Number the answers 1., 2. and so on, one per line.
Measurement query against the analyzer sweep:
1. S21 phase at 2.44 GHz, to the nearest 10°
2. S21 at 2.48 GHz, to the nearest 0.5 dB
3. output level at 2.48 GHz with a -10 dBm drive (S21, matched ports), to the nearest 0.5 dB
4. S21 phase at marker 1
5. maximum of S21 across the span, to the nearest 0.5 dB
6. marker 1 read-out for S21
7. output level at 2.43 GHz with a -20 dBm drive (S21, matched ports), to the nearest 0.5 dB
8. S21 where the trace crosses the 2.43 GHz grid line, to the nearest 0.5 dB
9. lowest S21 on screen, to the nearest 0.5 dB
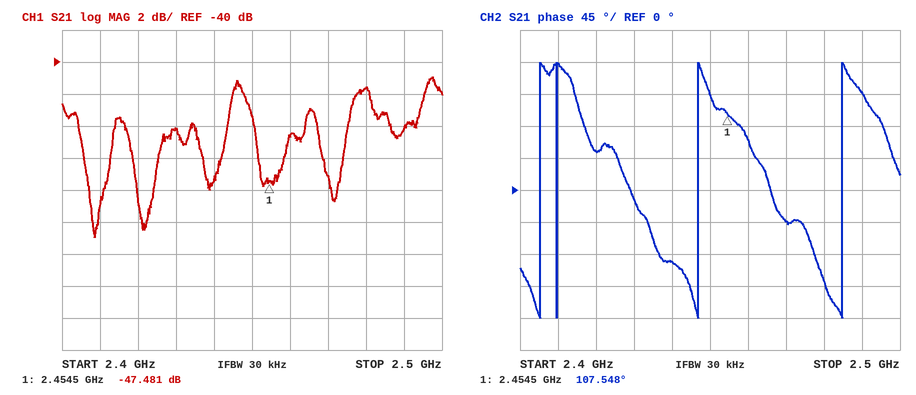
1. -100°
2. -41.5 dB
3. -51.5 dBm
4. 107.548°
5. -41.0 dB
6. -47.481 dB
7. -64.0 dBm
8. -44.0 dB
9. -51.0 dB
